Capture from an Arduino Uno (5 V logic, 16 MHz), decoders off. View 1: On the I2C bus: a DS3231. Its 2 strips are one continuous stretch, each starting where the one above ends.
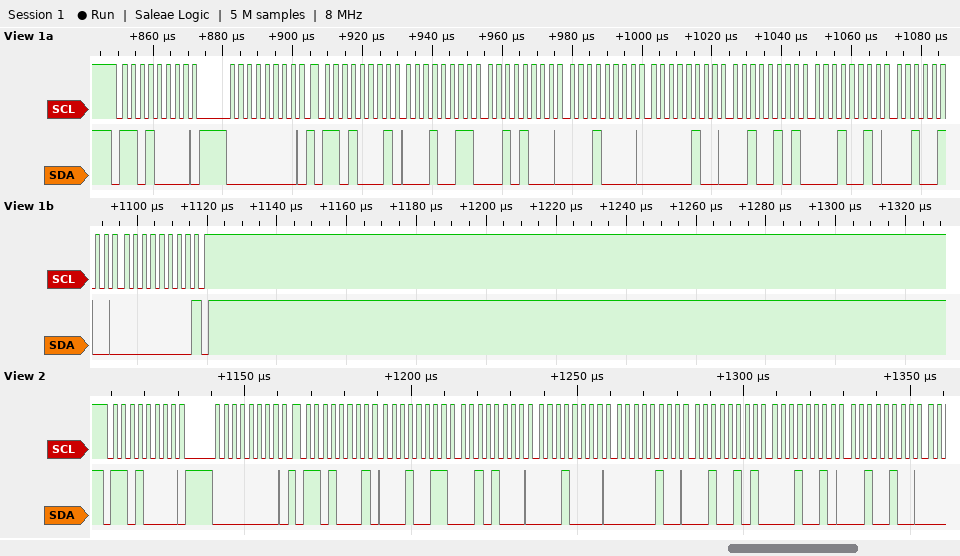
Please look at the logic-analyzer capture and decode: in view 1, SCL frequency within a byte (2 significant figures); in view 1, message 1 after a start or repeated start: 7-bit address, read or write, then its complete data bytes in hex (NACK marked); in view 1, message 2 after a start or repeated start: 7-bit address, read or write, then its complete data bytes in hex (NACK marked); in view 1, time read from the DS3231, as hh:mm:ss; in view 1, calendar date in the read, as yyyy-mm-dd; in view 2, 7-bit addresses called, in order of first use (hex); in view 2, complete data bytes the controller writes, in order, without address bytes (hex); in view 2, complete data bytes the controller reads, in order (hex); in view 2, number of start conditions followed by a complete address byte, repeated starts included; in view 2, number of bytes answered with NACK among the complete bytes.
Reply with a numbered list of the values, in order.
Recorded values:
1. 400 kHz
2. 0x68 write: 00
3. 0x68 read: 13 28 10 04 25 12 24 00 NACK
4. 10:28:13
5. 2024-12-25
6. 0x68
7. 00
8. 13 28 10 04 25 12 24
9. 2
10. 0
